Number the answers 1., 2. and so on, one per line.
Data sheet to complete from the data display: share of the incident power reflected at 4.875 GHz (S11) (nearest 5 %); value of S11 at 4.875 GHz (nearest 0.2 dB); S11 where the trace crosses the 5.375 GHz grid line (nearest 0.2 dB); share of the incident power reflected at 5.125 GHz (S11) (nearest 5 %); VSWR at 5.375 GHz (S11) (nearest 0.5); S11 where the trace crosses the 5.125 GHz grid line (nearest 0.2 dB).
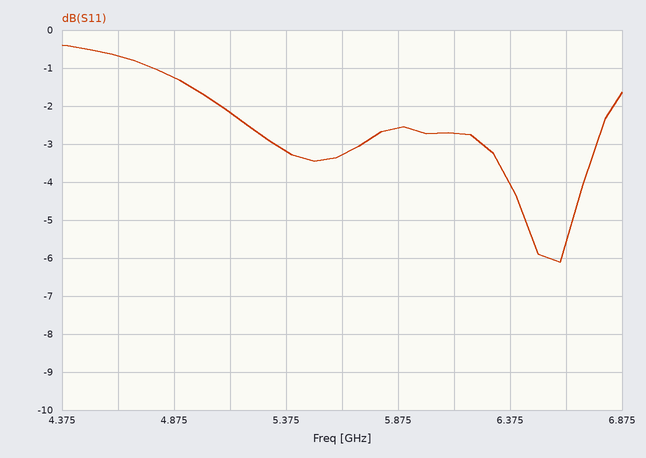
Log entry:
1. 75 %
2. -1.2 dB
3. -3.2 dB
4. 60 %
5. 5.5
6. -2.2 dB
